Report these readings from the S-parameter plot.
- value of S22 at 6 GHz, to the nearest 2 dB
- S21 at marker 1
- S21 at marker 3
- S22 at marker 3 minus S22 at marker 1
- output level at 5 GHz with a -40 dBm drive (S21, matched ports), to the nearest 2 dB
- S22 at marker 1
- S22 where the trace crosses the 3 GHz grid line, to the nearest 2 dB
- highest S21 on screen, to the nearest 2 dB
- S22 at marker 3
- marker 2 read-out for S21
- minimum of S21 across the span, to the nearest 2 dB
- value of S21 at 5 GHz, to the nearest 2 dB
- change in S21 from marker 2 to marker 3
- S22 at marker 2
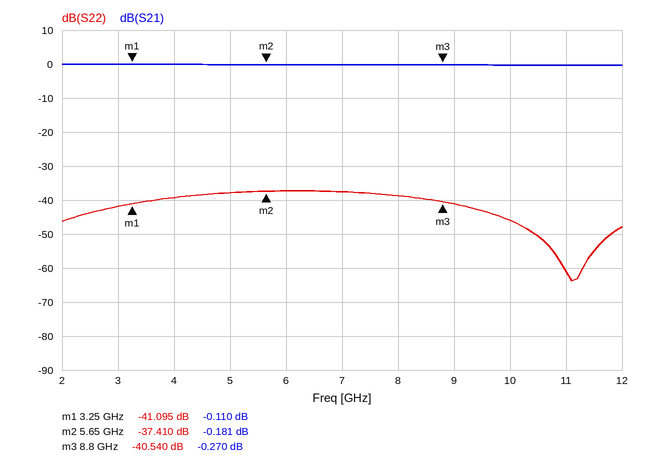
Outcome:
-38 dB
-0.110 dB
-0.270 dB
0.555 dB
-40 dBm
-41.095 dB
-42 dB
0 dB
-40.540 dB
-0.181 dB
0 dB
0 dB
-0.089 dB
-37.410 dB
